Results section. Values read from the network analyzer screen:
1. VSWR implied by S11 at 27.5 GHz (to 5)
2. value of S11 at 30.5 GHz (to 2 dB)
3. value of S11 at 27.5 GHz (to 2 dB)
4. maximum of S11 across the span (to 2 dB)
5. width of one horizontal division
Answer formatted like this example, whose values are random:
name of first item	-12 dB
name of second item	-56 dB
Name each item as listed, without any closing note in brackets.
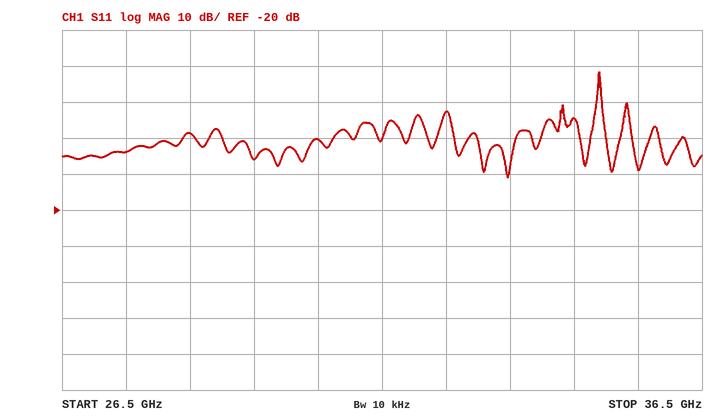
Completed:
VSWR implied by S11 at 27.5 GHz	5
value of S11 at 30.5 GHz	0 dB
value of S11 at 27.5 GHz	-4 dB
maximum of S11 across the span	18 dB
width of one horizontal division	1 GHz
